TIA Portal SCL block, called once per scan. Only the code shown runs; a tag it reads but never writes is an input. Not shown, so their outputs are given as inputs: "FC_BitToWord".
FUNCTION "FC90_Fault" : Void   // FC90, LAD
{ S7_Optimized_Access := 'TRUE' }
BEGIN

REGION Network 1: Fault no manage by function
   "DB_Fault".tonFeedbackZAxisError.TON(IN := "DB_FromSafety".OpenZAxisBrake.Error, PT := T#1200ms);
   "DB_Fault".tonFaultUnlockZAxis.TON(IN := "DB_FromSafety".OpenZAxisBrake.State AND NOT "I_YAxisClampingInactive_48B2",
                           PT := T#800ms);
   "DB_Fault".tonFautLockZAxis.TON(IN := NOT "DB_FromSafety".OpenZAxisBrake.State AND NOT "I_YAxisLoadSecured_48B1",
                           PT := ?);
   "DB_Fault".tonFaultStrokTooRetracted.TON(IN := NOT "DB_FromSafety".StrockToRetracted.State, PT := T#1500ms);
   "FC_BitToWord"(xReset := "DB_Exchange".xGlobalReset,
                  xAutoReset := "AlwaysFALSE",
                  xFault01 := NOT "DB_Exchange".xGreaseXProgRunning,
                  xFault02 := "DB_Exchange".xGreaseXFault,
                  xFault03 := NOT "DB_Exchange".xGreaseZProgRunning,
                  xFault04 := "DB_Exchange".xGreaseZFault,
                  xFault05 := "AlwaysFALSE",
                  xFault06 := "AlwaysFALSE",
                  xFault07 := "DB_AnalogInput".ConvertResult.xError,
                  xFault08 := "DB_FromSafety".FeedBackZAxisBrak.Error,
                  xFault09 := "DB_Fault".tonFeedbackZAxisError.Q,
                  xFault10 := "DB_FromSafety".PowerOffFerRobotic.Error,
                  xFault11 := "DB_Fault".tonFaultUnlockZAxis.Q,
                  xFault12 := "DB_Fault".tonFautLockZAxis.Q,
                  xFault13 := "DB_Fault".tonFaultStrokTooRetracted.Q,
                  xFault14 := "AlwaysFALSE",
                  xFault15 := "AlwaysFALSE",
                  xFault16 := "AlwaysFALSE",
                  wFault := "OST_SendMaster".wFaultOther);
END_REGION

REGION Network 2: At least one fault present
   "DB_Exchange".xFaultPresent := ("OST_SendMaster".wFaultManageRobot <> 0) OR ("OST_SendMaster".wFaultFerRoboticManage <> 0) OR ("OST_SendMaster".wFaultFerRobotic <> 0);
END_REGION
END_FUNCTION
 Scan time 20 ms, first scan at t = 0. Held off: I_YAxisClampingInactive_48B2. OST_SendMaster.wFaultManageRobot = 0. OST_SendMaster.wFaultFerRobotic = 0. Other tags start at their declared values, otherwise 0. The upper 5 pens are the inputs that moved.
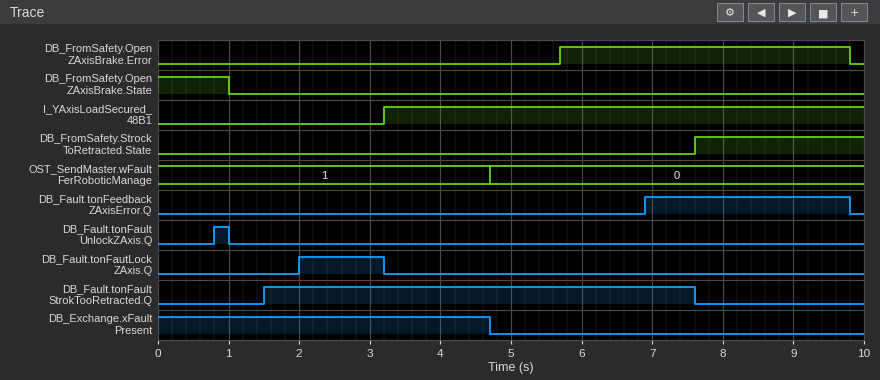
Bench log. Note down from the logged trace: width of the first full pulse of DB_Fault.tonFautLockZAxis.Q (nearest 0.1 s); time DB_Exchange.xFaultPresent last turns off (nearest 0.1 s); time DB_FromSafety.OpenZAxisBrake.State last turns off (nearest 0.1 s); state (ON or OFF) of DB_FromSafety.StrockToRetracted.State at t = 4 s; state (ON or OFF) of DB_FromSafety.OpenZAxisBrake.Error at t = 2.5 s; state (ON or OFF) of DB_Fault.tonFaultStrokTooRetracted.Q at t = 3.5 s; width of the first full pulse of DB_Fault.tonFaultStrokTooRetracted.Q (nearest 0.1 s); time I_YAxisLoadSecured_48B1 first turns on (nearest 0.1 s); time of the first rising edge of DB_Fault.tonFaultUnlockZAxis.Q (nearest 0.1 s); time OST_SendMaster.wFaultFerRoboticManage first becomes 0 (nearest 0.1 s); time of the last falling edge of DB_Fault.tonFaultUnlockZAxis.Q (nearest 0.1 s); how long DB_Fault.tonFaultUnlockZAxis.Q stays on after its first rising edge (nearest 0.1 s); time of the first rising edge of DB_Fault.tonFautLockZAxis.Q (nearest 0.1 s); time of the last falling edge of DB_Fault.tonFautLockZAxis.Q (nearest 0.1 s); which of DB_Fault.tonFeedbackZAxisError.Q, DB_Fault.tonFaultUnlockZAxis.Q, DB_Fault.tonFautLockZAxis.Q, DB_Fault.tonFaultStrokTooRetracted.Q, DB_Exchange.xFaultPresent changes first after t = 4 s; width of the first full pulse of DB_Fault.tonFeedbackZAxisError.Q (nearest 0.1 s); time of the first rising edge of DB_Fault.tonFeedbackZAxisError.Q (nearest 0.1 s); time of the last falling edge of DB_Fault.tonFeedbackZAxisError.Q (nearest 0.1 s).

1.2 s
4.7 s
1.0 s
OFF
OFF
ON
6.1 s
3.2 s
0.8 s
4.7 s
1.0 s
0.2 s
2.0 s
3.2 s
DB_Exchange.xFaultPresent
2.9 s
6.9 s
9.8 s
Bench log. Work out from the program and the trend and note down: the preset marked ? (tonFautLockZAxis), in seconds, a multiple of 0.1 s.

1.0 s
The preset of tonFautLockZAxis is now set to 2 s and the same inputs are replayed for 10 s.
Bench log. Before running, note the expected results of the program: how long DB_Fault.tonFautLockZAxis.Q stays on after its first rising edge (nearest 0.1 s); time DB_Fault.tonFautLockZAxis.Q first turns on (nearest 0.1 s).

0.2 s
3.0 s
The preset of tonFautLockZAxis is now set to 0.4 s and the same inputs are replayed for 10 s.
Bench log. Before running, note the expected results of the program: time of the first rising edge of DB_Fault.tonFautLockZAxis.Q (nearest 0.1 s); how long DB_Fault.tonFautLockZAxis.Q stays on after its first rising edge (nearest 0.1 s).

1.4 s
1.8 s
